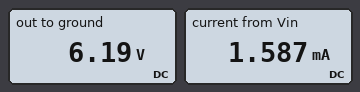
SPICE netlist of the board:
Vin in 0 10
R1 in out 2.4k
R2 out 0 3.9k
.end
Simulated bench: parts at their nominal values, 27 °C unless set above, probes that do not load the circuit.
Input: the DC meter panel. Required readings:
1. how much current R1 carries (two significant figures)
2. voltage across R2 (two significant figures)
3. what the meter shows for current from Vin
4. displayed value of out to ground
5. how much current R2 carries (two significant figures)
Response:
1.6 mA
6.2 V
1.587 mA
6.19 V
1.6 mA
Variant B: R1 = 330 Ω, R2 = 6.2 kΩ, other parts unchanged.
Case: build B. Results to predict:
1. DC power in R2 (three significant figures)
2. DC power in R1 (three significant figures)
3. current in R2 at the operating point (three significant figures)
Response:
14.5 mW
774 µW
1.53 mA
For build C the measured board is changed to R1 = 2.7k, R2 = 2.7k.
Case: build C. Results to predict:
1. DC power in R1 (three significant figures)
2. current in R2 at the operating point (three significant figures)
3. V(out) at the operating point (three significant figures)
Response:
9.26 mW
1.85 mA
5.00 V
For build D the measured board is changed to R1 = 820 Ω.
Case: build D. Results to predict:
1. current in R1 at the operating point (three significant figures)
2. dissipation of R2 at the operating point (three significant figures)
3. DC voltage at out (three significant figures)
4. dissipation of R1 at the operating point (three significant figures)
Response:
2.12 mA
17.5 mW
8.26 V
3.68 mW
